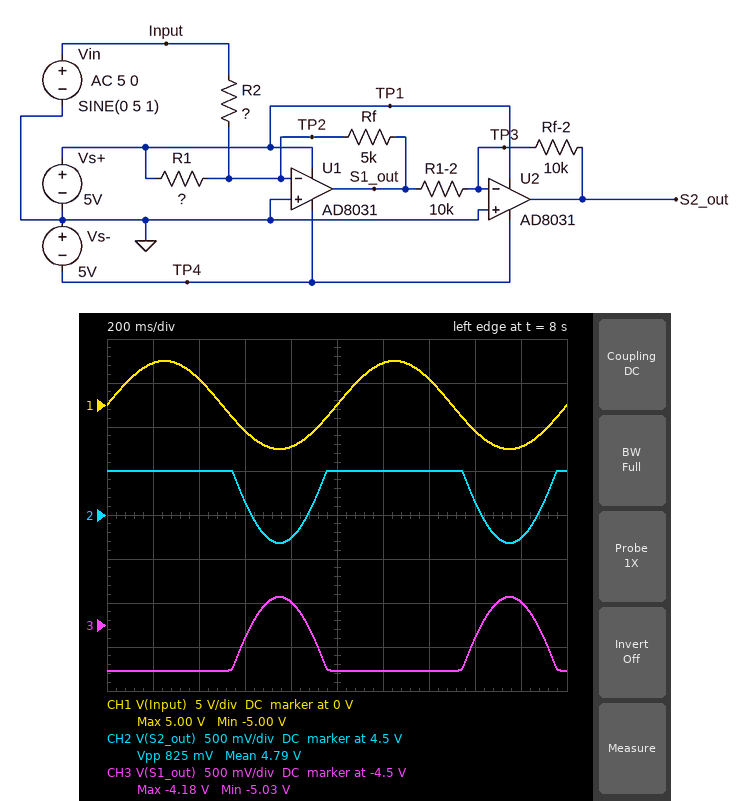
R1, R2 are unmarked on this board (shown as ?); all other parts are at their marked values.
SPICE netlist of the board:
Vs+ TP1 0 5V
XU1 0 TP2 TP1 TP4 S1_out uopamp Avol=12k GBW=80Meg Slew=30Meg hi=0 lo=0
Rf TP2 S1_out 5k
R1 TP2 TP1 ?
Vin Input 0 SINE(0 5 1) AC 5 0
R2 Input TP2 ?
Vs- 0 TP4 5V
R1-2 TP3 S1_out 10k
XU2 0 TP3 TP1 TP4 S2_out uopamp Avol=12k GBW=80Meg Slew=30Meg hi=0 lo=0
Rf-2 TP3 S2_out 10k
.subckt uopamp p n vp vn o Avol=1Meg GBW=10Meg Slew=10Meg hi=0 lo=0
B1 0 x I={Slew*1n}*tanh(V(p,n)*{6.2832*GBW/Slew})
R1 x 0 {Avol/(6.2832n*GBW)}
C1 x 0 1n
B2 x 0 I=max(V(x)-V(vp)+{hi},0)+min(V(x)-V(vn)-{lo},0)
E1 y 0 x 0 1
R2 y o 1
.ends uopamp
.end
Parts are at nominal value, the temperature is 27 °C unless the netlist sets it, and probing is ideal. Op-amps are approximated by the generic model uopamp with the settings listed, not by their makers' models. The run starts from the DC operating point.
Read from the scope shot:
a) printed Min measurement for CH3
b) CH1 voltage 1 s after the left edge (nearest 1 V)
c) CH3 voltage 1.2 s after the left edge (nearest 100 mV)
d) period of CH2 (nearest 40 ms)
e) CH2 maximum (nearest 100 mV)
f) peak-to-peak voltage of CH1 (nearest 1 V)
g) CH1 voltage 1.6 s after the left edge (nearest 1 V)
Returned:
-5.03 V
0 V
-5.0 V
1.00 s
5.0 V
10 V
-3 V
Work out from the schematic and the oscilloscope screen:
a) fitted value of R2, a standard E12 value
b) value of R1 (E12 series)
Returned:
22 kΩ
4.7 kΩ
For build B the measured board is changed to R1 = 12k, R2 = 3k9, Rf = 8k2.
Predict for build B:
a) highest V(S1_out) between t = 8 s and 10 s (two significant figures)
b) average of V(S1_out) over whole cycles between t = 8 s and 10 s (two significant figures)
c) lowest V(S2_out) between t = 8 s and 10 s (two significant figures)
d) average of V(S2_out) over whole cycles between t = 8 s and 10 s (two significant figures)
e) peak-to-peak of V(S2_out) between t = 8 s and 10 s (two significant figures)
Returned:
5.0 V
-1.1 V
-5.0 V
1.1 V
10 V
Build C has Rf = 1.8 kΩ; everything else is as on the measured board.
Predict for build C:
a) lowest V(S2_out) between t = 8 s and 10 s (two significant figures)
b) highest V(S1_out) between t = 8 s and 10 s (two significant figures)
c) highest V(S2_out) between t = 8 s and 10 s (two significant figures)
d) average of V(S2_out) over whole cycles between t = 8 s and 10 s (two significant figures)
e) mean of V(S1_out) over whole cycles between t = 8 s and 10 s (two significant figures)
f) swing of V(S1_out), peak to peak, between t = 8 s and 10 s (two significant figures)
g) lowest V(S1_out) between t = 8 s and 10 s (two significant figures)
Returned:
1.5 V
-1.5 V
2.3 V
1.9 V
-1.9 V
820 mV
-2.3 V
